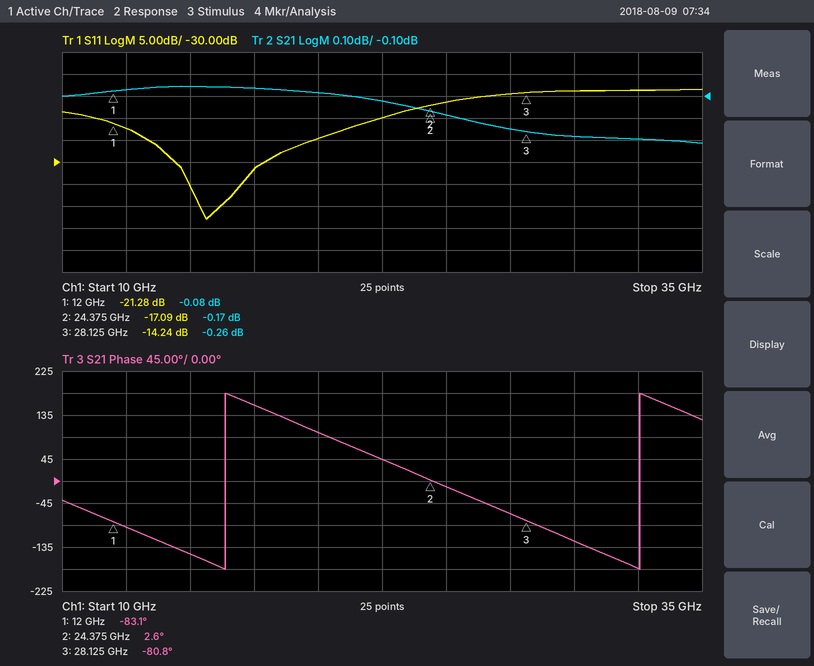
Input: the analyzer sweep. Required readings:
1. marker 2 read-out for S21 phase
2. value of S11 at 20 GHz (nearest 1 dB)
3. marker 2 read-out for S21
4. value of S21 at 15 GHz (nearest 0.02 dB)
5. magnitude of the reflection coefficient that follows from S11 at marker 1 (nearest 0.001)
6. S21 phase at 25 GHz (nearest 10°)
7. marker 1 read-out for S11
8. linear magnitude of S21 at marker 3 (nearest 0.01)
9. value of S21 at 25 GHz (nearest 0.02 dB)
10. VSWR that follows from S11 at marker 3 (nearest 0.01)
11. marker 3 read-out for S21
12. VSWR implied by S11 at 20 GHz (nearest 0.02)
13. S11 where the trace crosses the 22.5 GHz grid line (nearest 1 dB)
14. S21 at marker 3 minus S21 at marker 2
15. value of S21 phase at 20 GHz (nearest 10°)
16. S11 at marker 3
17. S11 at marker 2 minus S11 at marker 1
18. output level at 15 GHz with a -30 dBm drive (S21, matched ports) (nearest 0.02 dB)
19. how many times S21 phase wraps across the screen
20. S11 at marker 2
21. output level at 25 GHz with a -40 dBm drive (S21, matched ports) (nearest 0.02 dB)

2.6°
-25 dB
-0.17 dB
-0.06 dB
0.086
-10°
-21.28 dB
0.97
-0.18 dB
1.48
-0.26 dB
1.12
-20 dB
-0.09 dB
100°
-14.24 dB
4.19 dB
-30.06 dBm
2
-17.09 dB
-40.18 dBm
